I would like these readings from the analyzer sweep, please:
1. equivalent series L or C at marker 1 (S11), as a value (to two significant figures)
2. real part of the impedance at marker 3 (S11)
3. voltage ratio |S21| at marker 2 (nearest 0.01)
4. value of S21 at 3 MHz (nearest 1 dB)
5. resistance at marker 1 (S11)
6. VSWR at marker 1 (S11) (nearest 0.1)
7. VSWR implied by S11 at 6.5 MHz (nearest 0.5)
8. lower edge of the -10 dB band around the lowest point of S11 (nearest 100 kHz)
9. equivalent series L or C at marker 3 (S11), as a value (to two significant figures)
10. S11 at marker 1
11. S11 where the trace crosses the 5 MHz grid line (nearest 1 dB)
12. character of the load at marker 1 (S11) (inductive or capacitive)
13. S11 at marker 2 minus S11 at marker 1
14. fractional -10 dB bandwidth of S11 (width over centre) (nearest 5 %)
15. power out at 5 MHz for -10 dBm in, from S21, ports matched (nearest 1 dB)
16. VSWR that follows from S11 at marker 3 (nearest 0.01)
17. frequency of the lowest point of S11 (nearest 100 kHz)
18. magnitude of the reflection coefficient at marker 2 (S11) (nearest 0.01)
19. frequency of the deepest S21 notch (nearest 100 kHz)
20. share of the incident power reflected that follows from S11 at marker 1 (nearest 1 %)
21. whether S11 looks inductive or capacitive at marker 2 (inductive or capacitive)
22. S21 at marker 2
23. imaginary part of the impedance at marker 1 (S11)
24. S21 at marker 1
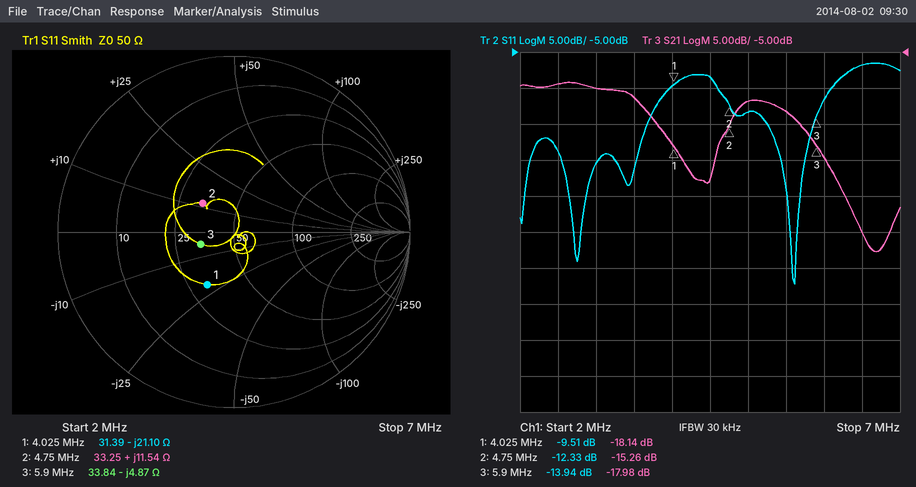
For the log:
1.9 nF
33.84 Ω
0.17
-10 dB
31.39 Ω
2.0
2.5
4.6 MHz
5.5 nF
-9.51 dB
-13 dB
capacitive
-2.82 dB
30 %
-22 dBm
1.50
5.6 MHz
0.24
6.7 MHz
11 %
inductive
-15.26 dB
-21.10 Ω
-18.14 dB
